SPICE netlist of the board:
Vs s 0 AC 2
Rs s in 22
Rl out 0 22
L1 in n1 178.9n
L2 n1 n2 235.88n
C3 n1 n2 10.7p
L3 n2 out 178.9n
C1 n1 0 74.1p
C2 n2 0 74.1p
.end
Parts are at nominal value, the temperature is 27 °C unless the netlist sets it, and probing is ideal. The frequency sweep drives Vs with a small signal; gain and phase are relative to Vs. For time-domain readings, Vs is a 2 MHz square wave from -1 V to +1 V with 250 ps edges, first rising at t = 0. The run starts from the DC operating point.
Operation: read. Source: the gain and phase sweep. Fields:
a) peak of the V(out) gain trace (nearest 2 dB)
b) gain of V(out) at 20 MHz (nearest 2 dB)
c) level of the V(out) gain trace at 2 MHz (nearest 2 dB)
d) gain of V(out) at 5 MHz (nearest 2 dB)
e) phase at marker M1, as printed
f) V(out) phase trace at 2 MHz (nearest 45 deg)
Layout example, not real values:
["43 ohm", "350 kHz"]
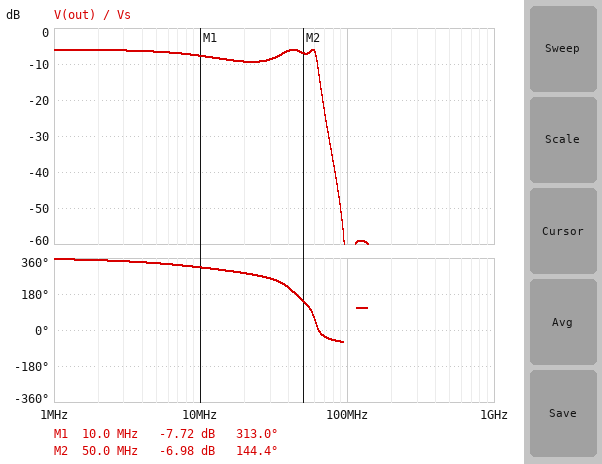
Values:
["-6 dB", "-10 dB", "-6 dB", "-6 dB", "313.0 deg", "360 deg"]
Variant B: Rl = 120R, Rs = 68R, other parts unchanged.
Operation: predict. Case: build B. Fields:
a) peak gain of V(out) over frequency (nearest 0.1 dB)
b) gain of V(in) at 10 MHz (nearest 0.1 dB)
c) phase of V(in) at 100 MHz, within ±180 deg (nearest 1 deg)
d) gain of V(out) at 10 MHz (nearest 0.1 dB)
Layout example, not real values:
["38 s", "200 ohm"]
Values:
["-3.9 dB", "-5.1 dB", "37 deg", "-4.0 dB"]
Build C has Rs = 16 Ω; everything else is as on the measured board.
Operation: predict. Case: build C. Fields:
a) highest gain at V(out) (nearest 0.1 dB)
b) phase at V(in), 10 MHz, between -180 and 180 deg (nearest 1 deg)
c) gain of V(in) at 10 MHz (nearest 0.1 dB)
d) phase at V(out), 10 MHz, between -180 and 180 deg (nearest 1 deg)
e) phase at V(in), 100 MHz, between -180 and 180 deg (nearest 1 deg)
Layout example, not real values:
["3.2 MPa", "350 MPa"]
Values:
["-4.7 dB", "12 deg", "-2.0 dB", "-50 deg", "10 deg"]
